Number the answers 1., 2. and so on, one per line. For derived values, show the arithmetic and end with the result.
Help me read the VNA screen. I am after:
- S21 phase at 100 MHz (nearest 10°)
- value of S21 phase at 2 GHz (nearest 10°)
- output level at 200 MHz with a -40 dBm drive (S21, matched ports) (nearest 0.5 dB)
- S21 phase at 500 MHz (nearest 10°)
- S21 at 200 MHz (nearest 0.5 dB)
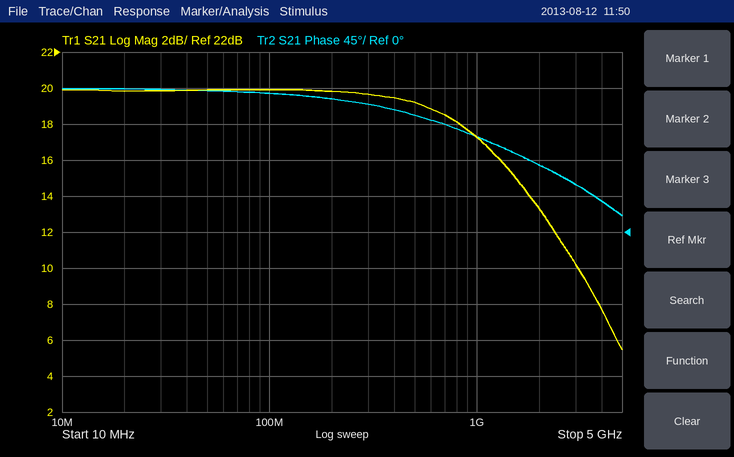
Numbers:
1. 170°
2. 80°
3. -40 dBm + (20.0 dB) = -20.0 dBm
4. 150°
5. 20.0 dB
